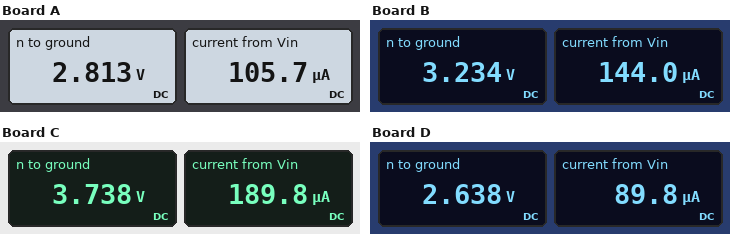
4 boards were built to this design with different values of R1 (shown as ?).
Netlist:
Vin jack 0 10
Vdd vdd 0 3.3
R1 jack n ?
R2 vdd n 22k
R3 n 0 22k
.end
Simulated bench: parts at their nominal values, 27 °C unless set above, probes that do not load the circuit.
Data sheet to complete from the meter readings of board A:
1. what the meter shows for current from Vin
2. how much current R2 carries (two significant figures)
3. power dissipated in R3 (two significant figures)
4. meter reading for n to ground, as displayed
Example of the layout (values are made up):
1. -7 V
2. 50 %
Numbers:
1. 105.7 µA
2. 22 µA
3. 360 µW
4. 2.813 V
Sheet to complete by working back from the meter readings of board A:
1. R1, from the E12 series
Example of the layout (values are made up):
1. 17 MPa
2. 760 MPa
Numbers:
1. 68 kΩ
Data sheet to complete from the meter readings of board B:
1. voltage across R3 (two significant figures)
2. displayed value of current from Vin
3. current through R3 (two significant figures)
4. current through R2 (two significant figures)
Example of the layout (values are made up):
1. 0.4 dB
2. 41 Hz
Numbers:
1. 3.2 V
2. 144.0 µA
3. 150 µA
4. 3.0 µA
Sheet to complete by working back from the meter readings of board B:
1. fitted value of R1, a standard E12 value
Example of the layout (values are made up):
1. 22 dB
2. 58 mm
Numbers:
1. 47 kΩ
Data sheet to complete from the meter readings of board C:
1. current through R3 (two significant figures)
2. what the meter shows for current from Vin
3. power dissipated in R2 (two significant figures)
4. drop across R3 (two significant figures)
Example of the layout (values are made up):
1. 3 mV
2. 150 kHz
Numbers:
1. 170 µA
2. 189.8 µA
3. 8.7 µW
4. 3.7 V
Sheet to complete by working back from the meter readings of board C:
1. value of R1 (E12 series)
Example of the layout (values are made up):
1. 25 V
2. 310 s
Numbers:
1. 33 kΩ
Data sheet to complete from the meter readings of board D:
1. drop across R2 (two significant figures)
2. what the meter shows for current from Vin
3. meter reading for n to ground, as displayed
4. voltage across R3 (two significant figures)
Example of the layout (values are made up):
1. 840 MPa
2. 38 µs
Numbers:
1. 660 mV
2. 89.8 µA
3. 2.638 V
4. 2.6 V
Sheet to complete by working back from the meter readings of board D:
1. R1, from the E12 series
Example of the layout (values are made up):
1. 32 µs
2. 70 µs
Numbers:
1. 82 kΩ
